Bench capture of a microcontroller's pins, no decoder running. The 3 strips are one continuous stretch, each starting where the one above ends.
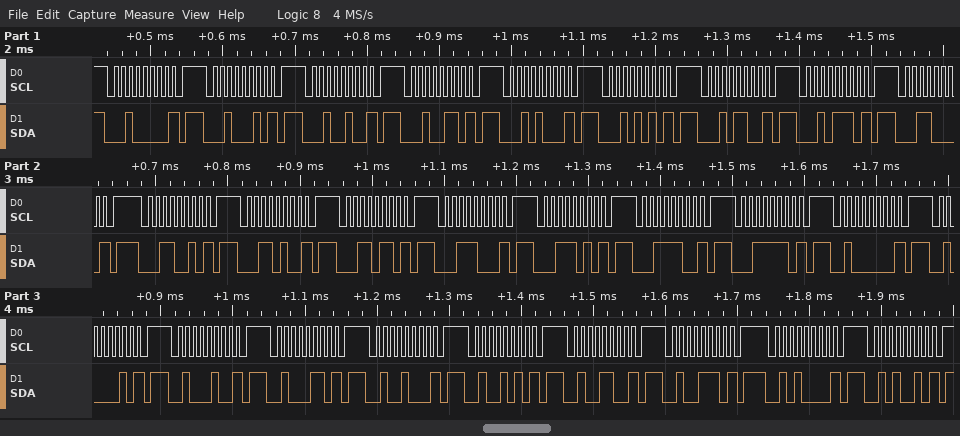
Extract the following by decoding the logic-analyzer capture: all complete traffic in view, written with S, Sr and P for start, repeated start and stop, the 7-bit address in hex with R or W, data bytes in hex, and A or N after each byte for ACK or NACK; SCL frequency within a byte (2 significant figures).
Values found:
S 10W N P S 11W N P S 12W N P S 13W N P S 14W N P S 15W N P S 16W N P S 17W N P S 18W N P S 19W N P S 1AW N P S 1BW N P S 1CW N P S 1DW N P S 1EW N P S 1FW N P S 20W N P S 21W N P S 22W N P S 23W N P S 24W N P S 25W N P S 26W N P S 27W N P S 28W N P S 29W N P
100 kHz
